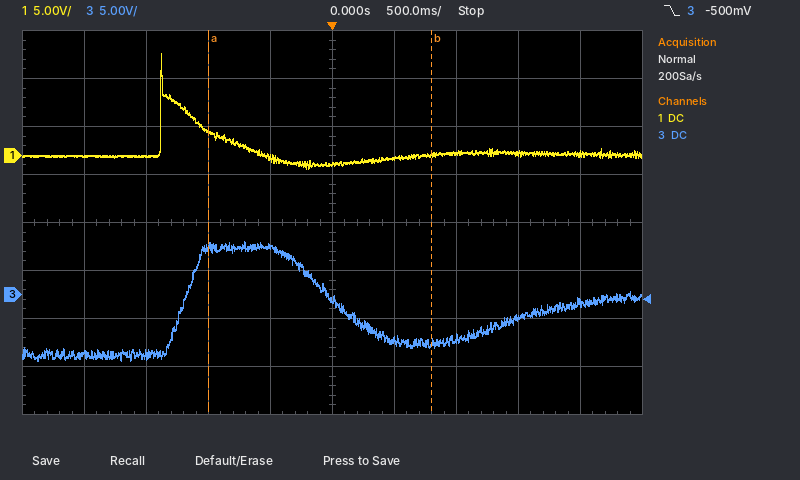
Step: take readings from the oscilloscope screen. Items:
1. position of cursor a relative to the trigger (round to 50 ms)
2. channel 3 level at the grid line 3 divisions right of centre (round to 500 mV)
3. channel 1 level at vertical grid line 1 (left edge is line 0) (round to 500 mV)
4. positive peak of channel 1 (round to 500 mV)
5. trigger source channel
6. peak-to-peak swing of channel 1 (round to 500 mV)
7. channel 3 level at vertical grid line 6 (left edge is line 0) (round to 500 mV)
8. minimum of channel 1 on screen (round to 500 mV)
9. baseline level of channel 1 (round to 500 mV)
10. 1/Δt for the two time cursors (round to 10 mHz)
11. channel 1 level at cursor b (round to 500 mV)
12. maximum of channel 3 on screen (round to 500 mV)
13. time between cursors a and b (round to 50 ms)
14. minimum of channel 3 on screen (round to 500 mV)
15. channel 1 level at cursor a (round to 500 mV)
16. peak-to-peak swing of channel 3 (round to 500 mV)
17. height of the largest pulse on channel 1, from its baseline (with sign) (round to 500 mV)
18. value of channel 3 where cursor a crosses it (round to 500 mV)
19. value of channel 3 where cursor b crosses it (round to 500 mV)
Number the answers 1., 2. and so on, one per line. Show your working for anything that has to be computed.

1. -1.00 s
2. -2.5 V
3. 0.0 V
4. 10.5 V
5. channel 3
6. 10.5 V − (-1.5 V) = 12.0 V
7. -5.0 V
8. -1.5 V
9. 0.0 V
10. 1 / 1.80 s ≈ 560 mHz
11. 0.0 V
12. 5.5 V
13. 1.80 s
14. -7.0 V
15. 2.5 V
16. 5.5 V − (-7.0 V) = 12.5 V
17. 10.5 V − (0.0 V) = +10.5 V
18. 5.0 V
19. -5.0 V
